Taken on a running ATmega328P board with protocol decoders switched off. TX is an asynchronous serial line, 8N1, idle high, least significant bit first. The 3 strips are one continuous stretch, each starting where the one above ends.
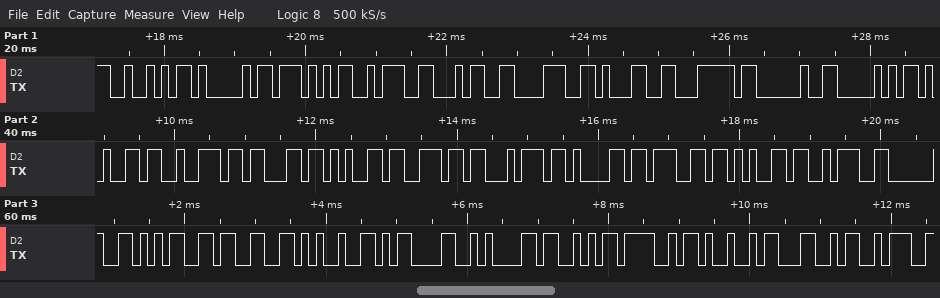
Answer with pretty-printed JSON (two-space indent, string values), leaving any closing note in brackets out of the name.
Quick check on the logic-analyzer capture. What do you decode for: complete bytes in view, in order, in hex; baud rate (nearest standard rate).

{
  "complete bytes in view, in order, in hex": "52 41 57 3A 34 38 31 7C 20 50 65 72 63 65 6E 74 61 67 65 3A 20 35 33 25 0D 0A 53 4F 49 4C 3A",
  "baud rate": "9600 baud"
}
